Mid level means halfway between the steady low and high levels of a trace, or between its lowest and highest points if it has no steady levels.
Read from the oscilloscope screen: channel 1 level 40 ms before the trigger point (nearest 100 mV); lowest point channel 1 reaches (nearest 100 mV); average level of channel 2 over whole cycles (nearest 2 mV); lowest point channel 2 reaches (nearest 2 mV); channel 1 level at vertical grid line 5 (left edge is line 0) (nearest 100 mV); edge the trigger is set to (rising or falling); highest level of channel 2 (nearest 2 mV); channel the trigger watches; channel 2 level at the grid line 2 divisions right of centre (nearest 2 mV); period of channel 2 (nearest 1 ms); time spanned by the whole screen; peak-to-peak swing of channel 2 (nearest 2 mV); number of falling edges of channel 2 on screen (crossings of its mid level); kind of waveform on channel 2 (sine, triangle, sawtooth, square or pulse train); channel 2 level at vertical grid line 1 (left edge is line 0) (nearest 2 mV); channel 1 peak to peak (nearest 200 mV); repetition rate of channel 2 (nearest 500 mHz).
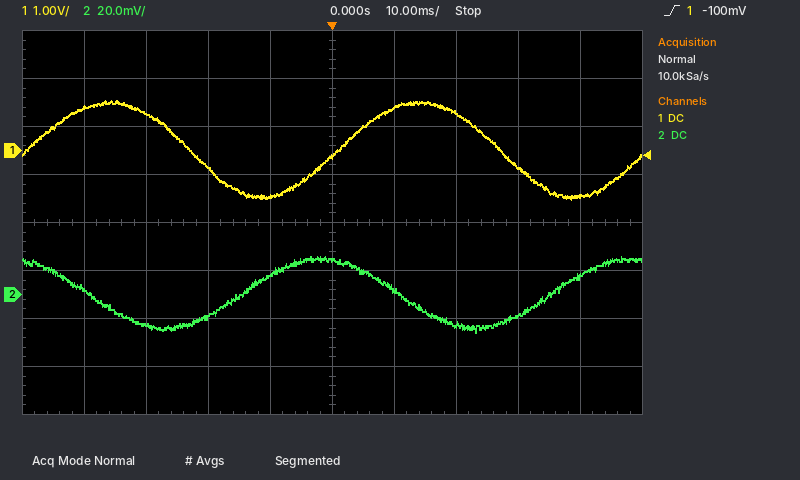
900 mV
-1.0 V
0 mV
-16 mV
-100 mV
rising
16 mV
channel 1
-12 mV
50 ms
100 ms
32 mV
2
sine
2 mV
2.0 V
20.0 Hz
